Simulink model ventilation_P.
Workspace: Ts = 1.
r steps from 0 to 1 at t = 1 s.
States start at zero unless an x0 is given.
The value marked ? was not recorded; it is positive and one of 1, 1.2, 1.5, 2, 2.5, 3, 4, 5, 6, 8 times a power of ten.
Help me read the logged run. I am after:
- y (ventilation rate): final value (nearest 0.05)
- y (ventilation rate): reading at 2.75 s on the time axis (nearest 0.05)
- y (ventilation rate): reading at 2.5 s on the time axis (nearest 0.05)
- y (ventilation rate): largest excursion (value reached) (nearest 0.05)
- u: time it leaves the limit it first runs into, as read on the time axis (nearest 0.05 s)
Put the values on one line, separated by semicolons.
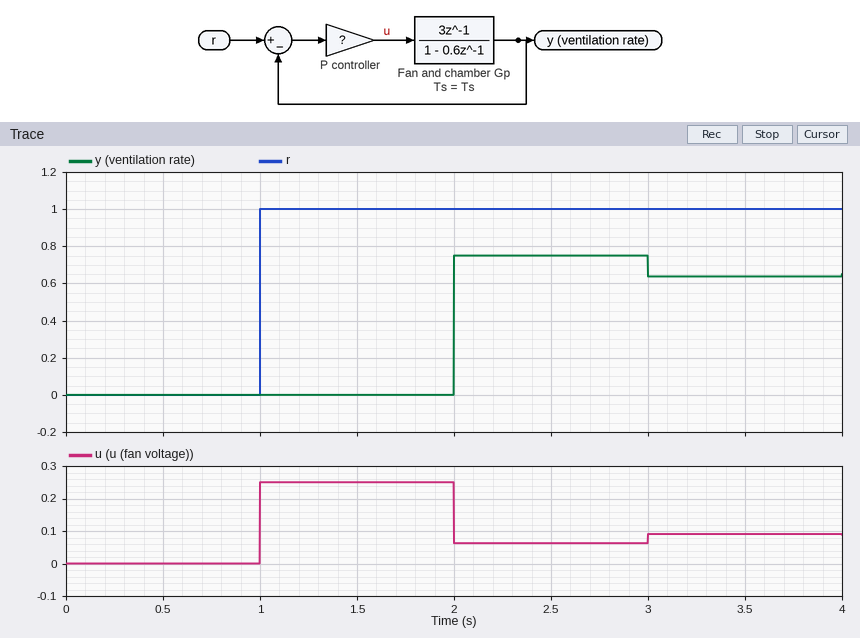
0.65; 0.75; 0.75; 0.75; 2.00 s
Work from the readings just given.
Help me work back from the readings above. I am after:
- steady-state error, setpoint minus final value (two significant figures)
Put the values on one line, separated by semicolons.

0.35
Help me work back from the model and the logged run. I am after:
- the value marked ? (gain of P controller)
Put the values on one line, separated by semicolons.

0.25
